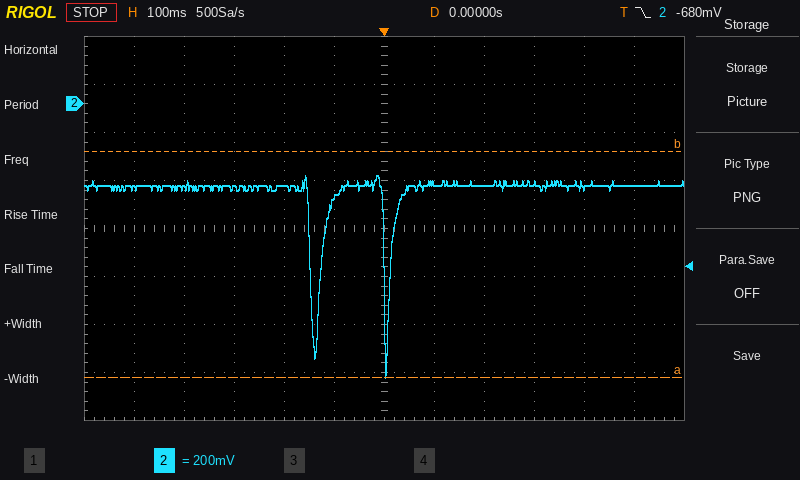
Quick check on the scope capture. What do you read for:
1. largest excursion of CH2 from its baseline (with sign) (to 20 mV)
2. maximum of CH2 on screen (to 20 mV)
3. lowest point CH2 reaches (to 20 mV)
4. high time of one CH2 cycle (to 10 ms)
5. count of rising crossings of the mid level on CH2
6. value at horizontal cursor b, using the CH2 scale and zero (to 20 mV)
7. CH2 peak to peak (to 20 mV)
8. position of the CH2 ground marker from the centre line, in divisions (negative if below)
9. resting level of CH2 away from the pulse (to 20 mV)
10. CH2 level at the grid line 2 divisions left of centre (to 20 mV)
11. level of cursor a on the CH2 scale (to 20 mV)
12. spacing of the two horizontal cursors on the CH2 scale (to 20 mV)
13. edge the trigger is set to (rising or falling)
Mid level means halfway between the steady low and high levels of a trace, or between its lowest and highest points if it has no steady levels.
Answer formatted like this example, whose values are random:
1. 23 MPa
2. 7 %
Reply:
1. -800 mV
2. -300 mV
3. -1.14 V
4. 130 ms
5. 2
6. -200 mV
7. 840 mV
8. +2.6 div
9. -340 mV
10. -340 mV
11. -1.14 V
12. 940 mV
13. falling
